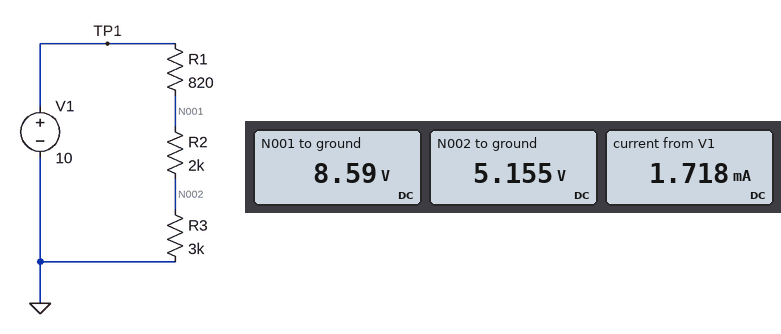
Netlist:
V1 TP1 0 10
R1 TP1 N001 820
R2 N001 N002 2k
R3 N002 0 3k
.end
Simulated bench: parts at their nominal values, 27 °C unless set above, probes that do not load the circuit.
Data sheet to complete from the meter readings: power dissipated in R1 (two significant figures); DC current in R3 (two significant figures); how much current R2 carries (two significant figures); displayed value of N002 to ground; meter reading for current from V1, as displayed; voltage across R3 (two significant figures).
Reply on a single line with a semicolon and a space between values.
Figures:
2.4 mW; 1.7 mA; 1.7 mA; 5.155 V; 1.718 mA; 5.2 V
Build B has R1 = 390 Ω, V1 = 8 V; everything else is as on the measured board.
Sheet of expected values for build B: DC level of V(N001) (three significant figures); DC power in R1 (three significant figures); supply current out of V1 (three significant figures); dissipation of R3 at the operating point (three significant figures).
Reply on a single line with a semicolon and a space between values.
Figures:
7.42 V; 859 µW; 1.48 mA; 6.61 mW
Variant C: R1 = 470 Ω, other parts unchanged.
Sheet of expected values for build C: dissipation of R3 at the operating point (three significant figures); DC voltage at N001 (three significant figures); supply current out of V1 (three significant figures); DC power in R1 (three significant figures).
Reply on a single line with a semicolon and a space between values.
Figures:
10.0 mW; 9.14 V; 1.83 mA; 1.57 mW
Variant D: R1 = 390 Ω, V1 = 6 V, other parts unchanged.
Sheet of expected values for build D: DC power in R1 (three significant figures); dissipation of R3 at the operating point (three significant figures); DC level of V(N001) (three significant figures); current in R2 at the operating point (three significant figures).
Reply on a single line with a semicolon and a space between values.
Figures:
483 µW; 3.72 mW; 5.57 V; 1.11 mA
